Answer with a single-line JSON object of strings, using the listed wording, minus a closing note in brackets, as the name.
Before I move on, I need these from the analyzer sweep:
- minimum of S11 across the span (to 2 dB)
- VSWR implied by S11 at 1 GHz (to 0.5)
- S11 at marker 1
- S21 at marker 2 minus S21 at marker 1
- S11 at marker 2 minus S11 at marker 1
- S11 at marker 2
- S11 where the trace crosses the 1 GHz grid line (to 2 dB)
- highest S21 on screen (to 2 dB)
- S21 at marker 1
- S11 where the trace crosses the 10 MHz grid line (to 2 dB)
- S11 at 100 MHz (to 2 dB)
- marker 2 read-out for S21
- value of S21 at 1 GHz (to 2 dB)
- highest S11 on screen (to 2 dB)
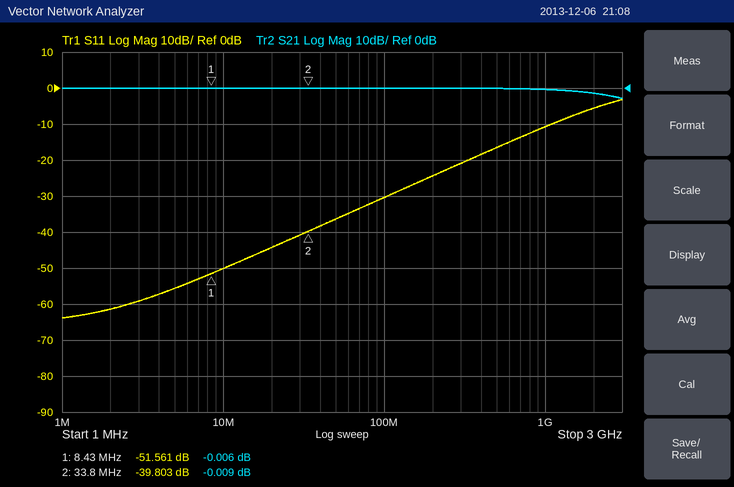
{"minimum of S11 across the span": "-64 dB", "VSWR implied by S11 at 1 GHz": "2.0", "S11 at marker 1": "-51.561 dB", "S21 at marker 2 minus S21 at marker 1": "-0.003 dB", "S11 at marker 2 minus S11 at marker 1": "11.758 dB", "S11 at marker 2": "-39.803 dB", "S11 where the trace crosses the 1 GHz grid line": "-10 dB", "highest S21 on screen": "0 dB", "S21 at marker 1": "-0.006 dB", "S11 where the trace crosses the 10 MHz grid line": "-50 dB", "S11 at 100 MHz": "-30 dB", "marker 2 read-out for S21": "-0.009 dB", "value of S21 at 1 GHz": "0 dB", "highest S11 on screen": "-4 dB"}
